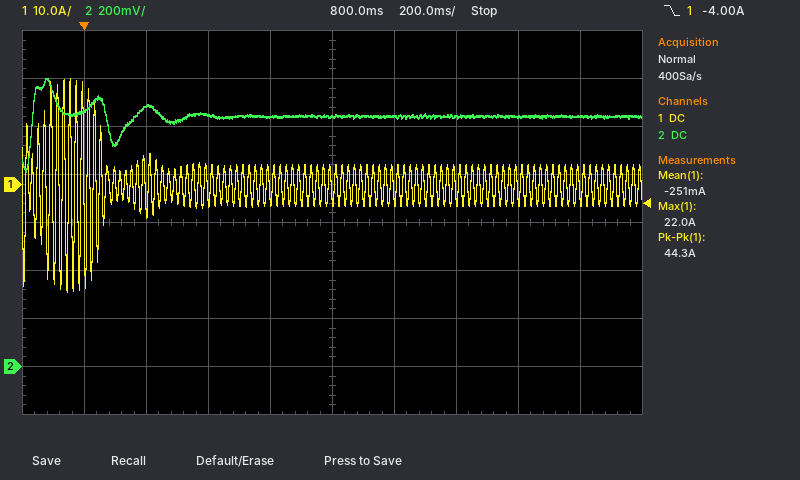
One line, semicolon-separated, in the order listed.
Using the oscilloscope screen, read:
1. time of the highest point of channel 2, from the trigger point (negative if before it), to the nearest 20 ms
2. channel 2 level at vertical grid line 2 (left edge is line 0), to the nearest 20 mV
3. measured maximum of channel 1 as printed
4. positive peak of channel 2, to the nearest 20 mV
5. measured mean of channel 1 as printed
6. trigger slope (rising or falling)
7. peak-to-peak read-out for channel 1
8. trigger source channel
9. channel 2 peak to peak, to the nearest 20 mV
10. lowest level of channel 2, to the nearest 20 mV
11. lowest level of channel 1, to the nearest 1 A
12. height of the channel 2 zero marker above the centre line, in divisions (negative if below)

-120 ms; 1.08 V; 22.0 A; 1.20 V; -251 mA; falling; 44.3 A; channel 1; 380 mV; 820 mV; -22 A; -3.0 div
